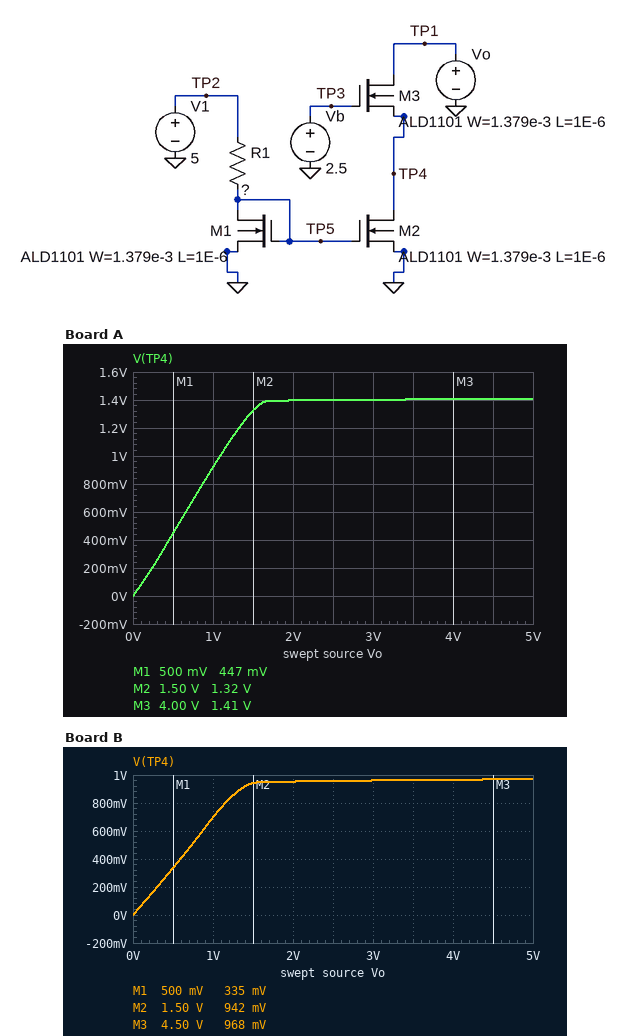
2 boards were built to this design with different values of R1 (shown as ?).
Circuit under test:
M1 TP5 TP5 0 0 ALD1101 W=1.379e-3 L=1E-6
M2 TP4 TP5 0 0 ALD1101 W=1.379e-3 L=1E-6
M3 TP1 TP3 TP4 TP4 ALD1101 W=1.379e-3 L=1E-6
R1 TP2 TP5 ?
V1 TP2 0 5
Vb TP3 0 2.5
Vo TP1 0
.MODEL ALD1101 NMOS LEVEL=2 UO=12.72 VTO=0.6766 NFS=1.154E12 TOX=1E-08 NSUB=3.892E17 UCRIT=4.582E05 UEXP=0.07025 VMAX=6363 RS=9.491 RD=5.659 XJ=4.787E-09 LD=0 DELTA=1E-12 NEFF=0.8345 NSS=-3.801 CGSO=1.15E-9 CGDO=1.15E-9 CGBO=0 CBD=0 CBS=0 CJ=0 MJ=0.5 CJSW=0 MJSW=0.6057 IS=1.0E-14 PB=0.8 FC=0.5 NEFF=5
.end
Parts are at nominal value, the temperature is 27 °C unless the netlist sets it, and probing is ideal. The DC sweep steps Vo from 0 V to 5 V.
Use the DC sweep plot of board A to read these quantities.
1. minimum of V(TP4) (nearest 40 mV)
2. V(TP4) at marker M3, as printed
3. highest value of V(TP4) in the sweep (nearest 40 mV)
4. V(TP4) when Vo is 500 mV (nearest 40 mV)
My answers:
0 V
1.41 V
1.40 V
440 mV
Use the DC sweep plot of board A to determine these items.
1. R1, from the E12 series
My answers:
10 kΩ
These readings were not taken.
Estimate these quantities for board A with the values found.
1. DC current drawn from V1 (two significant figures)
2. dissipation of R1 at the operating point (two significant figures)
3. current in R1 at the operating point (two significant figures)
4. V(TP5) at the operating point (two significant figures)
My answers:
390 µA
1.5 mW
390 µA
1.1 V
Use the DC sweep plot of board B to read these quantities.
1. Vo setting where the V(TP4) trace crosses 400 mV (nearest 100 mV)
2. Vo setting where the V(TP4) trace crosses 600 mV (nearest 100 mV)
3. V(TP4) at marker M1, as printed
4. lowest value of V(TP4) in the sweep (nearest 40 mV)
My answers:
600 mV
900 mV
335 mV
0 V
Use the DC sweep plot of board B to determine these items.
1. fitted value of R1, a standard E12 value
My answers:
2.2 kΩ
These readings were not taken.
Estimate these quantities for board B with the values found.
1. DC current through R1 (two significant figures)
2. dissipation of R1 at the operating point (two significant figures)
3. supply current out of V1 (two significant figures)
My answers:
1.6 mA
5.4 mW
1.6 mA
